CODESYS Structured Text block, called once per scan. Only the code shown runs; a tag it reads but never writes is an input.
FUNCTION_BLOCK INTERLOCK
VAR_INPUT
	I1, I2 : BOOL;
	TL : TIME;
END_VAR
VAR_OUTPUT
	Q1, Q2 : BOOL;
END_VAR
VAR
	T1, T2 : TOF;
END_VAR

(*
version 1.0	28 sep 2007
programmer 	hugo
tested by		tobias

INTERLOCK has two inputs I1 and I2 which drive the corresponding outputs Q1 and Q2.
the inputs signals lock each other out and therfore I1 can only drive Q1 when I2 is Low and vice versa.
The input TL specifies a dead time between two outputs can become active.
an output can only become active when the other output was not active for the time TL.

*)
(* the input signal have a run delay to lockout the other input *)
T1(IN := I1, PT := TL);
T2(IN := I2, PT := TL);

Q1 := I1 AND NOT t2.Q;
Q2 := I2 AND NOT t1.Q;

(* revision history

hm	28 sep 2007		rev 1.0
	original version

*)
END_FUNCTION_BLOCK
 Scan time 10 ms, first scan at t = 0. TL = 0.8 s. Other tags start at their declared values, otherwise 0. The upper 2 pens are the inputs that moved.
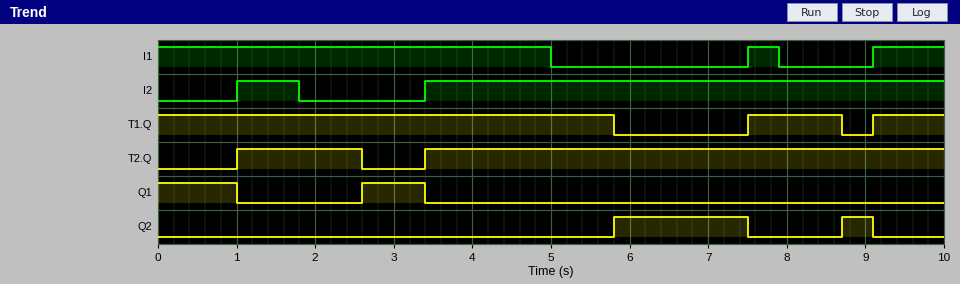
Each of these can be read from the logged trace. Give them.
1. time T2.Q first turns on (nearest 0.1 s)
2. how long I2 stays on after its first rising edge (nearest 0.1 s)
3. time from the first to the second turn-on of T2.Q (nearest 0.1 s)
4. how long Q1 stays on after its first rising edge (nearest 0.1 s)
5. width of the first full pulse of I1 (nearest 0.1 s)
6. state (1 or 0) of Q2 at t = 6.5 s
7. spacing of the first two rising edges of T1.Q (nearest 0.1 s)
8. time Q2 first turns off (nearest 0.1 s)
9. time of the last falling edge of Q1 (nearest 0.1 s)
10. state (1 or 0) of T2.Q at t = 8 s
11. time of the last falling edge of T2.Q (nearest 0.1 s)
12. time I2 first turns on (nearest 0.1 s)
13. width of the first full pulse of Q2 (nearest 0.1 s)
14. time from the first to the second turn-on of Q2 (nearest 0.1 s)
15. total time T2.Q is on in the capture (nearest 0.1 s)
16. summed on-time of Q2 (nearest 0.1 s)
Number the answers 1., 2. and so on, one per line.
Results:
1. 1.0 s
2. 0.8 s
3. 2.4 s
4. 0.8 s
5. 0.4 s
6. 1
7. 1.6 s
8. 7.5 s
9. 3.4 s
10. 1
11. 2.6 s
12. 1.0 s
13. 1.7 s
14. 2.9 s
15. 8.2 s
16. 2.1 s
